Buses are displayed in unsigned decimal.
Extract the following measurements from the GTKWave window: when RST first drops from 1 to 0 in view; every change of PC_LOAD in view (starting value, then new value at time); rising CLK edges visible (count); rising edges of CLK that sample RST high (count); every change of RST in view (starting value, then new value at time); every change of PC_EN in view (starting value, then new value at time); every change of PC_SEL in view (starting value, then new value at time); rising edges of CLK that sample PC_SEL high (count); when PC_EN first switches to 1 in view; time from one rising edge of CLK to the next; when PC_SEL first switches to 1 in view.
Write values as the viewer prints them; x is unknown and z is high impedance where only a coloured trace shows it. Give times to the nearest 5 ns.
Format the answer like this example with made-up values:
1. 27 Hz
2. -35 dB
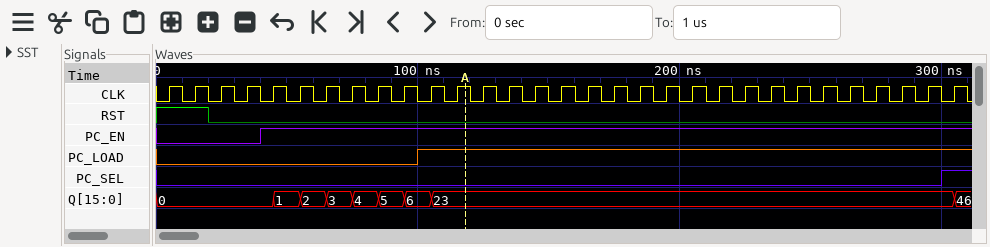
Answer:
1. 20 ns
2. 0, 1 at 100 ns
3. 31
4. 2
5. 1, 0 at 20 ns
6. 0, 1 at 40 ns
7. 0, 1 at 300 ns
8. 1
9. 40 ns
10. 10 ns
11. 300 ns
